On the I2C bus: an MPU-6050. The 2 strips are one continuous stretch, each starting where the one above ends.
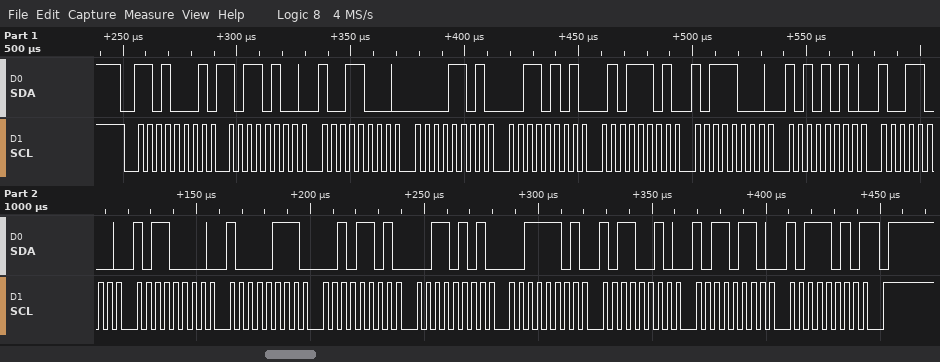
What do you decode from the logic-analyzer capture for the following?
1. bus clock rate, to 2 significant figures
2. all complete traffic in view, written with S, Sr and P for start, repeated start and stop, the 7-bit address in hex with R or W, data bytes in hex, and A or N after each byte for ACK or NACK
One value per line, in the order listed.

250 kHz
S 68R A B4 A 98 A 0D A 35 A 5D A B8 A AA A 98 A B0 A 87 A 2D A 35 A 3D A B2 A B6 A BA N P
